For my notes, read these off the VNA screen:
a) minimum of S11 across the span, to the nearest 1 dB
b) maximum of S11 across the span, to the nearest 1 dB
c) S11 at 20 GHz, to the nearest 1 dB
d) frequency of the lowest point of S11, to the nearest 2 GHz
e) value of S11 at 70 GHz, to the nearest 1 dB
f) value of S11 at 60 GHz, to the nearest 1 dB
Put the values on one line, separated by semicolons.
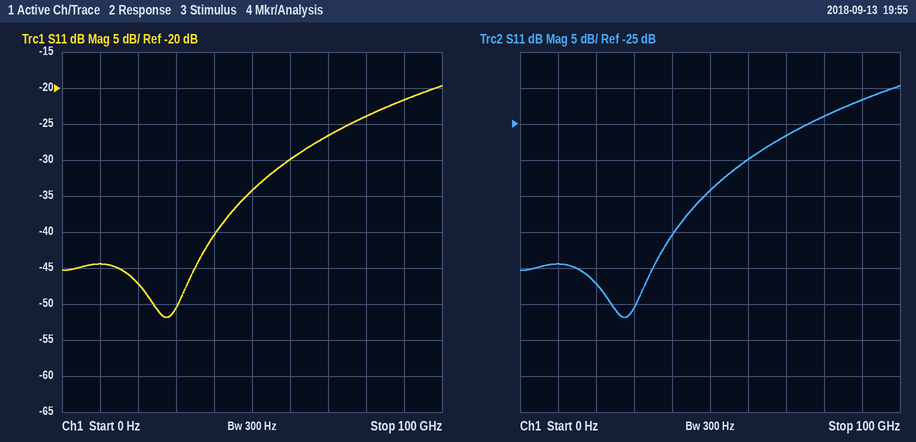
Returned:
-52 dB; -20 dB; -47 dB; 28 GHz; -27 dB; -30 dB
